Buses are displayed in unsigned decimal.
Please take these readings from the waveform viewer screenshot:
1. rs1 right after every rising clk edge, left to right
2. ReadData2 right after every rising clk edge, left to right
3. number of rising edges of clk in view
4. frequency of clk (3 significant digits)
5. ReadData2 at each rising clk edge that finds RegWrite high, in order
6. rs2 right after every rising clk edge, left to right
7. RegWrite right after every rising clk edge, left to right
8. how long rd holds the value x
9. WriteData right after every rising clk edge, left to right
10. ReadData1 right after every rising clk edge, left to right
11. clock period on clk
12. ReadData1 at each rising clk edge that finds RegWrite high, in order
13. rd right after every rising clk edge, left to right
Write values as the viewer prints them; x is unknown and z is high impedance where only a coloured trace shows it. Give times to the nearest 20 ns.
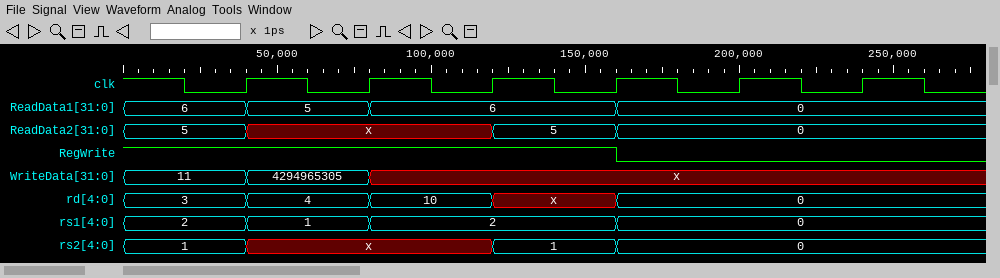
1, 2, 2, 0, 0, 0
x, x, 5, 0, 0, 0
6
25.0 MHz
5, x, x, 5
x, x, 1, 0, 0, 0
1 1 1 0 0 0
40 ns
4294965305, x, x, x, x, x
5, 6, 6, 0, 0, 0
40 ns
6, 5, 6, 6
4, 10, x, 0, 0, 0
